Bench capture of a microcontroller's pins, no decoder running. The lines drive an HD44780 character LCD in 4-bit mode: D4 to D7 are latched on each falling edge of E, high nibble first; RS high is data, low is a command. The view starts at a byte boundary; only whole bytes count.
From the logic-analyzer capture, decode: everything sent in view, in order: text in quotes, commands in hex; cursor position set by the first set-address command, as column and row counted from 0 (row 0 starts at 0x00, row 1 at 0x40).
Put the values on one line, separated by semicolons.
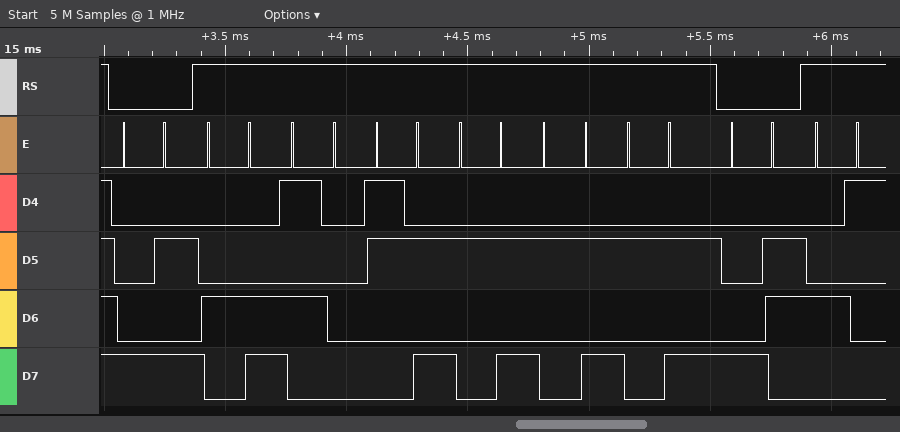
0x8A "LP:***" 0x86 "A"; column 10, row 0
